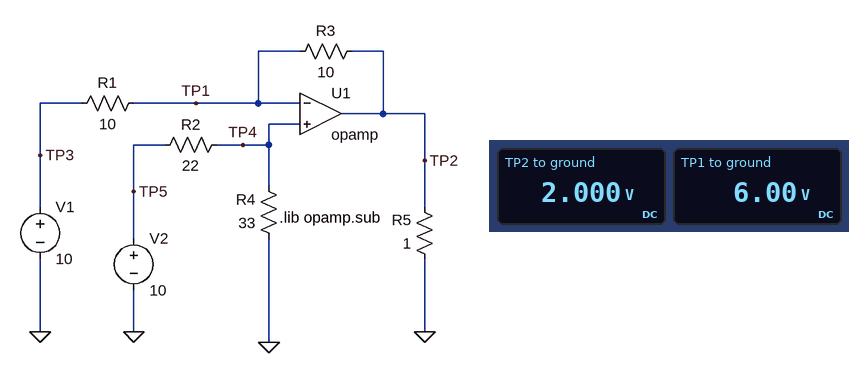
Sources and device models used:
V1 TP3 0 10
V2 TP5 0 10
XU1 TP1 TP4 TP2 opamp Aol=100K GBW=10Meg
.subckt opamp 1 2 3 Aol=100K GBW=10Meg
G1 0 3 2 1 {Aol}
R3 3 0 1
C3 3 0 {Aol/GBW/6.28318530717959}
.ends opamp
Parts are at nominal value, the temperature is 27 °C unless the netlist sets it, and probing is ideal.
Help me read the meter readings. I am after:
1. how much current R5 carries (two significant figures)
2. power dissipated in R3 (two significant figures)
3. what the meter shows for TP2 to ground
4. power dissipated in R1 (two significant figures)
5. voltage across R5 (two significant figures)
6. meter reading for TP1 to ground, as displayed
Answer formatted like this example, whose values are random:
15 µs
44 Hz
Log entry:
2.0 A
1.6 W
2.000 V
1.6 W
2.0 V
6.00 V
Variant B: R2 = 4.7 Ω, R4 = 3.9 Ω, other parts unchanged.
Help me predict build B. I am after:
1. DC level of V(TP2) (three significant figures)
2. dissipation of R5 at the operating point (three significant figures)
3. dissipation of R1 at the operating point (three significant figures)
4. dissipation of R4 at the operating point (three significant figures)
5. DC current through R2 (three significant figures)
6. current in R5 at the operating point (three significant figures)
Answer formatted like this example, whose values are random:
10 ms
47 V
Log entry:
-930 mV
865 mW
2.99 W
5.27 W
1.16 A
930 mA
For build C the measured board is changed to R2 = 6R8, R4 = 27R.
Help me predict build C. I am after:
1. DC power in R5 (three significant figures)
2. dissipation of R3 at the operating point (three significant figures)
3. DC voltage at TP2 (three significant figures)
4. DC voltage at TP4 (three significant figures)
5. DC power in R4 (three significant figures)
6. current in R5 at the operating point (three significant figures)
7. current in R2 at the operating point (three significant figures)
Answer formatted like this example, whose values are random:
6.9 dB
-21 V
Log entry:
35.7 W
405 mW
5.98 V
7.99 V
2.36 W
5.98 A
296 mA
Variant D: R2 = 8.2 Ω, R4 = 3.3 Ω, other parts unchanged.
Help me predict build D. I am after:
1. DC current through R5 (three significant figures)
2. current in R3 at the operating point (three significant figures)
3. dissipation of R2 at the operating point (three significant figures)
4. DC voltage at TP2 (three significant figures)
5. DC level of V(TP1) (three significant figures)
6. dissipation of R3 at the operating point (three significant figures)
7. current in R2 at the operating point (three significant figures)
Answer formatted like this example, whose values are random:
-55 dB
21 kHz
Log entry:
4.26 A
713 mA
6.20 W
-4.26 V
2.87 V
5.08 W
870 mA
